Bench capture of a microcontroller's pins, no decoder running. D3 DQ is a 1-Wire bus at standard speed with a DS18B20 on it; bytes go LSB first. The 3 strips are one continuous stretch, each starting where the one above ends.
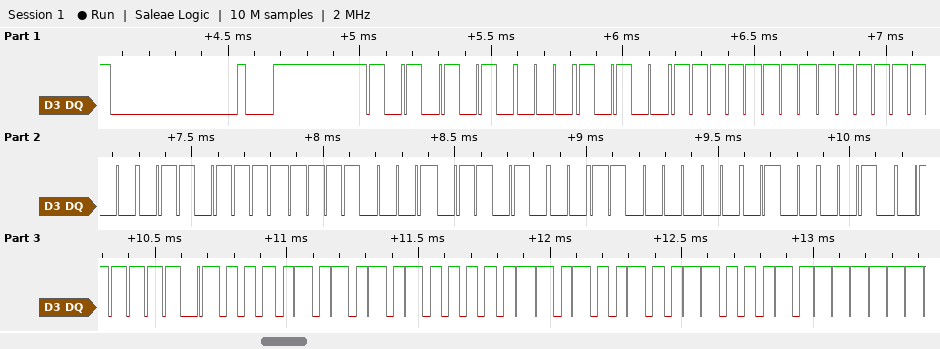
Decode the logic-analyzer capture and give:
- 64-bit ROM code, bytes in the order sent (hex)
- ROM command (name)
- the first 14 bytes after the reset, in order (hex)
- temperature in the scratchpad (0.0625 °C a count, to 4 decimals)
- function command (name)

28 FF 3F F6 8F 16 03 42
Match ROM
55 28 FF 3F F6 8F 16 03 42 BE 50 05 4B 46
85.0000 °C
Read Scratchpad
